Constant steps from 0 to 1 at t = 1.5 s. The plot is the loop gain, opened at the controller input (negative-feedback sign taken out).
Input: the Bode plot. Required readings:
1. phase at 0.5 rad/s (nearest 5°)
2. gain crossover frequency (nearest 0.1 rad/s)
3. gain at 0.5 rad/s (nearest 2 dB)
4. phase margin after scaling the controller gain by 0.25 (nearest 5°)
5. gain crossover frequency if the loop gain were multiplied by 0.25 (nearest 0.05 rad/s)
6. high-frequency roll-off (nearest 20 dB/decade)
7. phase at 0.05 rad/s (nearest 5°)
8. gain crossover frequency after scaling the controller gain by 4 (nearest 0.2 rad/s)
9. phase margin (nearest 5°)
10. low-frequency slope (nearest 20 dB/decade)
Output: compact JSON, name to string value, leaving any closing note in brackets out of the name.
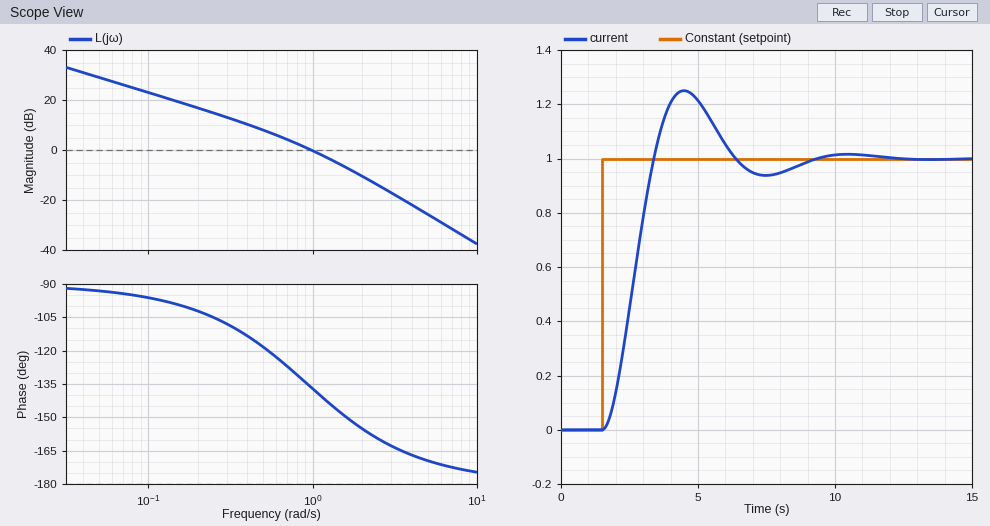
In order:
{"phase at 0.5 rad/s": "-120°", "gain crossover frequency": "1.0 rad/s", "gain at 0.5 rad/s": "8 dB", "phase margin after scaling the controller gain by 0.25": "70°", "gain crossover frequency if the loop gain were multiplied by 0.25": "0.35 rad/s", "high-frequency roll-off": "-40 dB/decade", "phase at 0.05 rad/s": "-95°", "gain crossover frequency after scaling the controller gain by 4": "2.2 rad/s", "phase margin": "45°", "low-frequency slope": "-20 dB/decade"}
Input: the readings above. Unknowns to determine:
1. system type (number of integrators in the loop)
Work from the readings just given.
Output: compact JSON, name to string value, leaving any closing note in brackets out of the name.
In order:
{"system type": "1"}
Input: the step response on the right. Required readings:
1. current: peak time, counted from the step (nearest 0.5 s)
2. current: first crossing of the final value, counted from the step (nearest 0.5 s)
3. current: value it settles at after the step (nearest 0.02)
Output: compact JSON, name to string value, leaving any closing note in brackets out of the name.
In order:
{"current: peak time, counted from the step": "3.0 s", "current: first crossing of the final value, counted from the step": "2.0 s", "current: value it settles at after the step": "1.00"}
